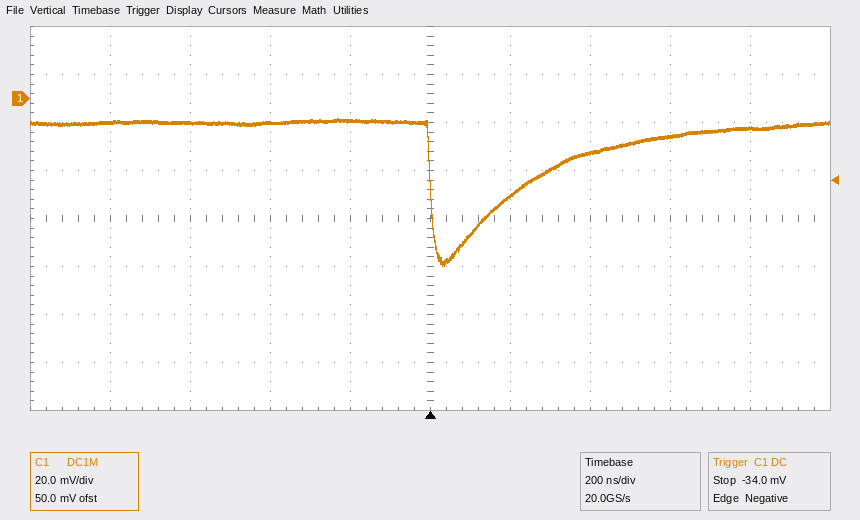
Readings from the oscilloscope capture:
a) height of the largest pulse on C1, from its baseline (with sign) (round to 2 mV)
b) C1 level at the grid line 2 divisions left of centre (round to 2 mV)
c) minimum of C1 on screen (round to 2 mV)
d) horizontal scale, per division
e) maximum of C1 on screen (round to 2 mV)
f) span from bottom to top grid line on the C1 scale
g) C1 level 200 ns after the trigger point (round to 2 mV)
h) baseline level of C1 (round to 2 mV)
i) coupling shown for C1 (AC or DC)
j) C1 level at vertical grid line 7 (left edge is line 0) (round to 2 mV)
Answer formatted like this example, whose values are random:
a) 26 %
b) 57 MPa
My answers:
a) -60 mV
b) -10 mV
c) -70 mV
d) 200 ns
e) -8 mV
f) 160 mV
g) -40 mV
h) -10 mV
i) DC
j) -22 mV
